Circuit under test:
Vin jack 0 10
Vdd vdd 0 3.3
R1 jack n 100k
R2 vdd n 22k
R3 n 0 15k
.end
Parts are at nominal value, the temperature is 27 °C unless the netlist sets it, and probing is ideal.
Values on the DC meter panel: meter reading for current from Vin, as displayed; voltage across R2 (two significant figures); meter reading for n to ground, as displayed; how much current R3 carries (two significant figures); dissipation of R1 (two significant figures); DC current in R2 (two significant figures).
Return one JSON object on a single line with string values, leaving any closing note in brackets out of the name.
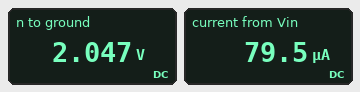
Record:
{"meter reading for current from Vin, as displayed": "79.5 µA", "voltage across R2": "1.3 V", "meter reading for n to ground, as displayed": "2.047 V", "how much current R3 carries": "140 µA", "dissipation of R1": "630 µW", "DC current in R2": "57 µA"}
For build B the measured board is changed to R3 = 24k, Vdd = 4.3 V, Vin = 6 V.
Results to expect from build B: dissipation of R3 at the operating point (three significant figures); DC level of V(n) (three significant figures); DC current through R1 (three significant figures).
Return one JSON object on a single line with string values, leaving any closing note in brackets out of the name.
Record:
{"dissipation of R3 at the operating point": "288 µW", "DC level of V(n)": "2.63 V", "DC current through R1": "33.7 µA"}
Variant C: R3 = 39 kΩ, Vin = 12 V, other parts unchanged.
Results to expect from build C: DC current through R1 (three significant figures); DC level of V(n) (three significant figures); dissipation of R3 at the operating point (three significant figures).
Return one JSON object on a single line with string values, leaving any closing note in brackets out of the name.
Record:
{"DC current through R1": "86.7 µA", "DC level of V(n)": "3.33 V", "dissipation of R3 at the operating point": "284 µW"}
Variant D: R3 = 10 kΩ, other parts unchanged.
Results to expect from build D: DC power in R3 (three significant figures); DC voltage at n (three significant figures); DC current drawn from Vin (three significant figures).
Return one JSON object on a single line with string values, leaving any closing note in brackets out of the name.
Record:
{"DC power in R3": "259 µW", "DC voltage at n": "1.61 V", "DC current drawn from Vin": "83.9 µA"}
